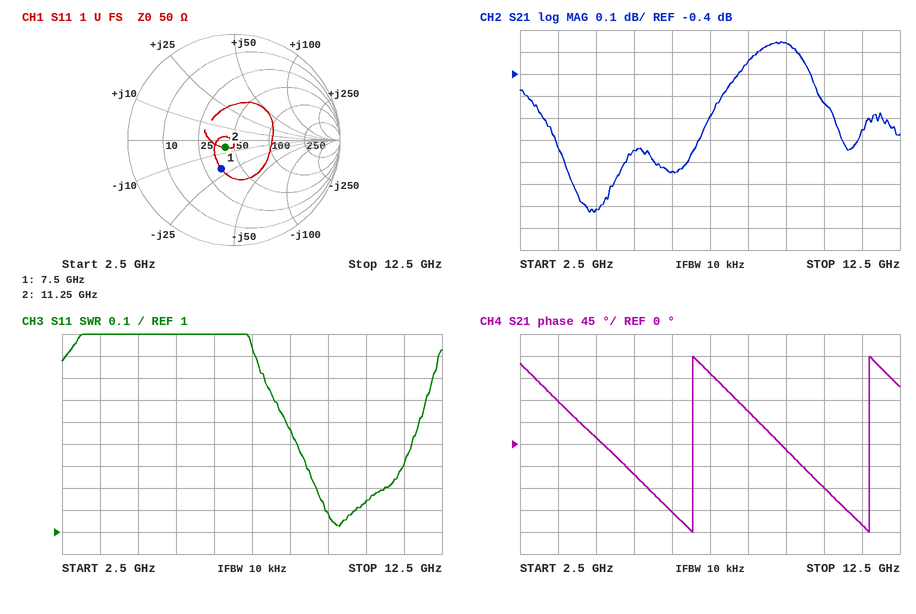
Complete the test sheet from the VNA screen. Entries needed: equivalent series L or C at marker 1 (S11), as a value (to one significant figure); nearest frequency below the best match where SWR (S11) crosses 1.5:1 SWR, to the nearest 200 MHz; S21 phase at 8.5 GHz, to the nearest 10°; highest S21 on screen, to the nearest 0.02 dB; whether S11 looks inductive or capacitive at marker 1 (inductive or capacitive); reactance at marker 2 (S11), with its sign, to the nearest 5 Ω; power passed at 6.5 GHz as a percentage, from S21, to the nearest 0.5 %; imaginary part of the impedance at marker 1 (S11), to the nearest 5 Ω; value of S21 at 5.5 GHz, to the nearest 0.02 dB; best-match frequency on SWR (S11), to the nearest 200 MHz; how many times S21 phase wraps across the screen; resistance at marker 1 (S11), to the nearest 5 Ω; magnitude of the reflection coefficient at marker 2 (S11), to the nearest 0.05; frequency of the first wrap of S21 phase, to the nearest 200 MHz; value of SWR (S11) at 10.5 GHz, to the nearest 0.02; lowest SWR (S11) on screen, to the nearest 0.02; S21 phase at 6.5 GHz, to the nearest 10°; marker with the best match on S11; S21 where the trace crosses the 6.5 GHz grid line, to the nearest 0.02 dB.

1 pF
8.4 GHz
70°
-0.26 dB
capacitive
-5 Ω
82.5 %
-20 Ω
-0.74 dB
9.8 GHz
2
35 Ω
0.10
7.0 GHz
1.14
1.02
-140°
marker 2
-0.84 dB
